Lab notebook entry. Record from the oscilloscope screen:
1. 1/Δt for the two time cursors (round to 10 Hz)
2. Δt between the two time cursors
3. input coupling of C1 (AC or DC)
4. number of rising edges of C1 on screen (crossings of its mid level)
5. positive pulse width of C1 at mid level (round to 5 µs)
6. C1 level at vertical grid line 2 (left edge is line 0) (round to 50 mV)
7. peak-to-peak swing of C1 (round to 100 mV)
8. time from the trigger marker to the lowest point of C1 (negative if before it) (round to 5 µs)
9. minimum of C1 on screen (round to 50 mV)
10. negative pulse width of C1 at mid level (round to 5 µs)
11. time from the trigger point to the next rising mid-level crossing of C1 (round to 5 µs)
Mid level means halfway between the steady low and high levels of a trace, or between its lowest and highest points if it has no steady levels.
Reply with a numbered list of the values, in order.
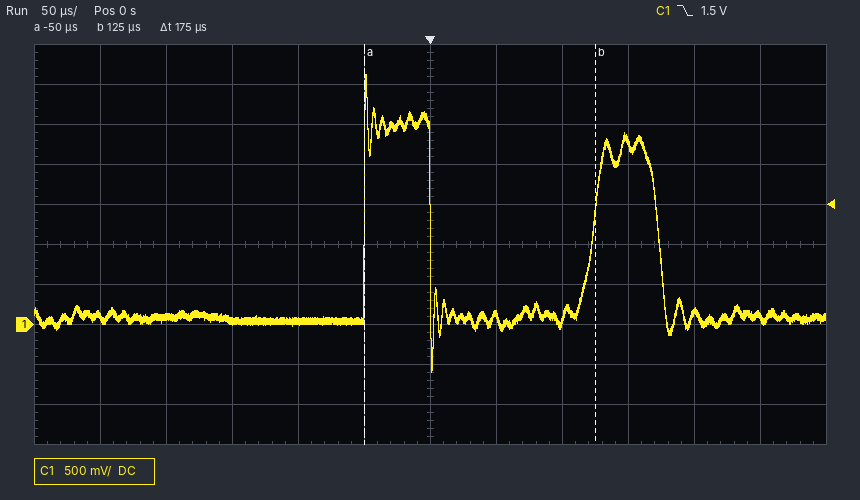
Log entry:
1. 5.71 kHz
2. 175 µs
3. DC
4. 2
5. 50 µs
6. 100 mV
7. 3.70 V
8. 0 µs
9. -600 mV
10. 125 µs
11. 125 µs
